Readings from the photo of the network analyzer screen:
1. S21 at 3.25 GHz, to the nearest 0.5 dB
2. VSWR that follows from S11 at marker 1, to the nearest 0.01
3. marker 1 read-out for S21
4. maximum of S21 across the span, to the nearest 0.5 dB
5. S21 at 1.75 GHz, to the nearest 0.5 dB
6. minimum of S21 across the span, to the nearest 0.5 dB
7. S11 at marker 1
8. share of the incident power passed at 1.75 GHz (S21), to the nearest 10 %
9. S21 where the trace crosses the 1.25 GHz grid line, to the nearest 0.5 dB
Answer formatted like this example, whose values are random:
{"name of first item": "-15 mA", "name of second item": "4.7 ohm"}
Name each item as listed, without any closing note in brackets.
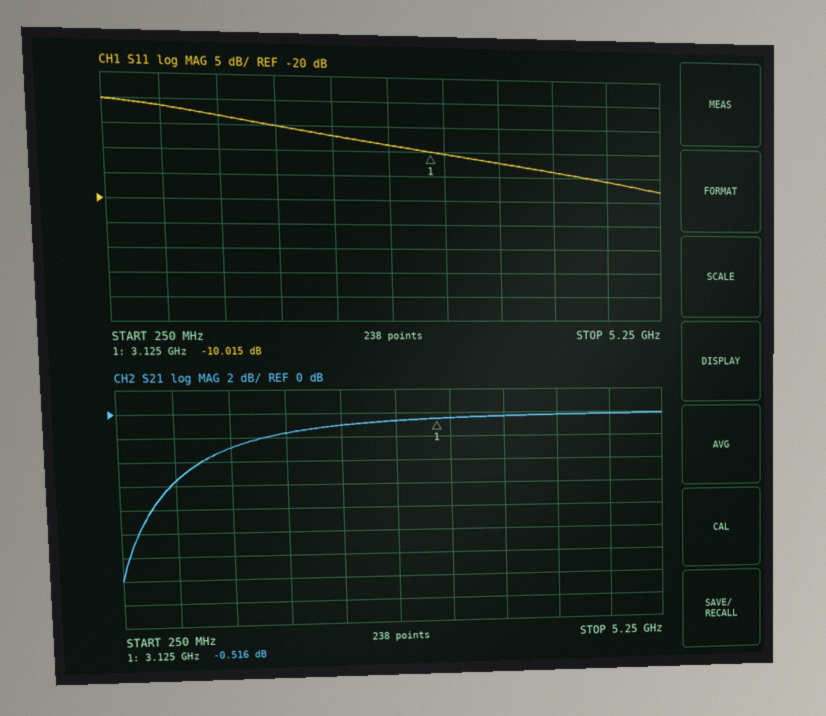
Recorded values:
{"S21 at 3.25 GHz, to the nearest 0.5 dB": "-0.5 dB", "VSWR that follows from S11 at marker 1, to the nearest 0.01": "1.92", "marker 1 read-out for S21": "-0.516 dB", "maximum of S21 across the span, to the nearest 0.5 dB": "0.0 dB", "S21 at 1.75 GHz, to the nearest 0.5 dB": "-1.5 dB", "minimum of S21 across the span, to the nearest 0.5 dB": "-14.0 dB", "S11 at marker 1": "-10.015 dB", "share of the incident power passed at 1.75 GHz (S21), to the nearest 10 %": "70 %", "S21 where the trace crosses the 1.25 GHz grid line, to the nearest 0.5 dB": "-3.0 dB"}
